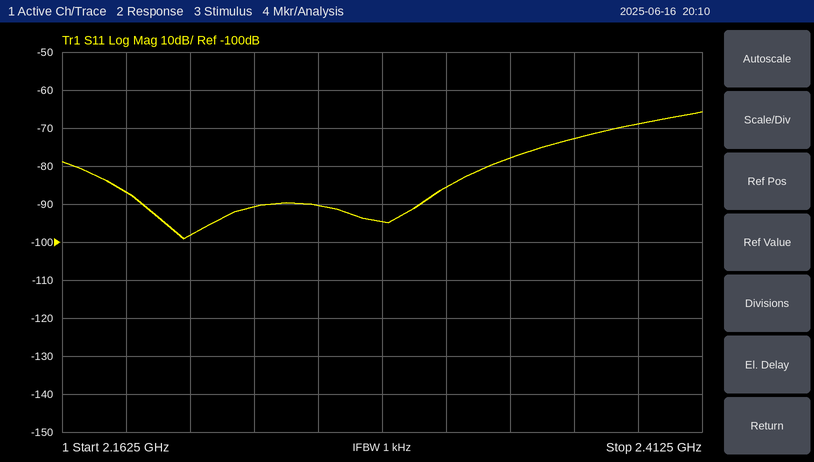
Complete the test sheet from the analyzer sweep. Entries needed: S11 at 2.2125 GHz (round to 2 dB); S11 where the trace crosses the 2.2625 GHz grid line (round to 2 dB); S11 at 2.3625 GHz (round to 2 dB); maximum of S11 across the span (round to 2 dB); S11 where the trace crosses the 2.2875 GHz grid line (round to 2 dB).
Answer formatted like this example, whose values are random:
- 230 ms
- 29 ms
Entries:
- -98 dB
- -90 dB
- -72 dB
- -66 dB
- -94 dB
